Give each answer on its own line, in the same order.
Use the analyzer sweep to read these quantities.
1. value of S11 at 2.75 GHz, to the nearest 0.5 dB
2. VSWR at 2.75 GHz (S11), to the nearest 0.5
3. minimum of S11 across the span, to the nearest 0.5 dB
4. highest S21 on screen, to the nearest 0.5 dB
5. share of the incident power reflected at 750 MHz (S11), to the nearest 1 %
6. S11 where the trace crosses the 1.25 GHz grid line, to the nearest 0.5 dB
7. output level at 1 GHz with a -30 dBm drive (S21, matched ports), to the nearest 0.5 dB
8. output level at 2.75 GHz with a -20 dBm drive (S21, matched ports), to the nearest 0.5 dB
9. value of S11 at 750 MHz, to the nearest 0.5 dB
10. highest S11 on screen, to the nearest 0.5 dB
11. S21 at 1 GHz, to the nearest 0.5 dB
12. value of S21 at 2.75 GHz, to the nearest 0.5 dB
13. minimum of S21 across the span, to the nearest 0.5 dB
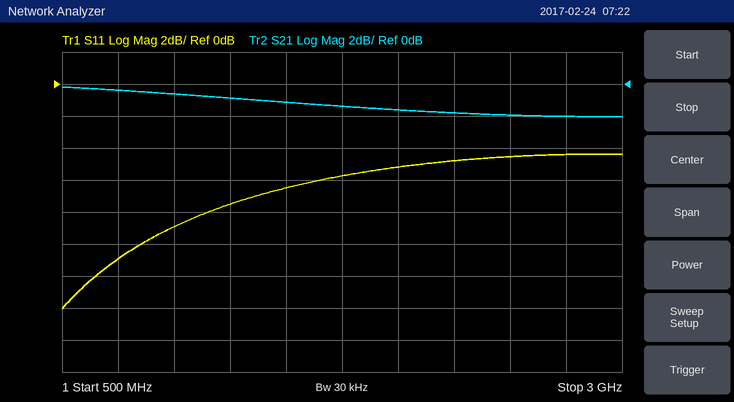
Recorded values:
-4.5 dB
4.0
-14.0 dB
0.0 dB
8 %
-7.5 dB
-30.5 dBm
-22.0 dBm
-11.0 dB
-4.5 dB
-0.5 dB
-2.0 dB
-2.0 dB
